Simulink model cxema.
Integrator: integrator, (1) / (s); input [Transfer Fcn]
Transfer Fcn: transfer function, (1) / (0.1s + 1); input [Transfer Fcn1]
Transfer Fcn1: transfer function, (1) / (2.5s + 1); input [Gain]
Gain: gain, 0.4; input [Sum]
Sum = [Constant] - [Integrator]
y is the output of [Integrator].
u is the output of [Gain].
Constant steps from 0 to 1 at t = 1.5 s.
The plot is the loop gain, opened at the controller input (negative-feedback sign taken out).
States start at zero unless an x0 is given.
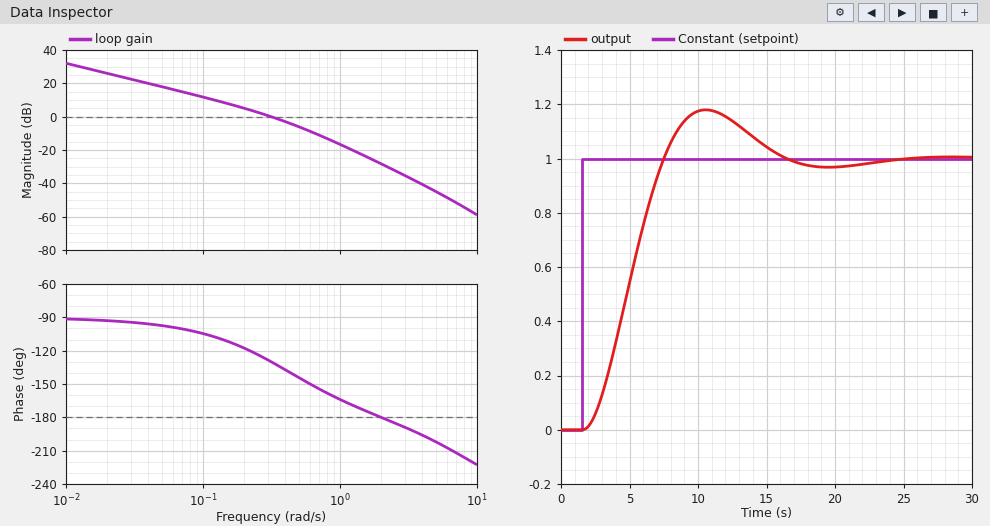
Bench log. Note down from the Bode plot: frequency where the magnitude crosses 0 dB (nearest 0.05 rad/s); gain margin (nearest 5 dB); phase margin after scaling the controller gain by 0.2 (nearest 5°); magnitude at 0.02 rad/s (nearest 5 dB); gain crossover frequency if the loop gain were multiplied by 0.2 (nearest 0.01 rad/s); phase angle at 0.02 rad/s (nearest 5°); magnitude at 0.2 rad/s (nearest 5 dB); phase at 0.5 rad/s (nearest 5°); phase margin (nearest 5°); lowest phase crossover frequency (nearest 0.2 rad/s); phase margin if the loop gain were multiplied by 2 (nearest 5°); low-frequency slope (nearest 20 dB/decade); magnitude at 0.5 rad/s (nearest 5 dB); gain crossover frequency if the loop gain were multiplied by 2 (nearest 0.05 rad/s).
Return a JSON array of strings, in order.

["0.30 rad/s", "30 dB", "80°", "25 dB", "0.08 rad/s", "-95°", "5 dB", "-145°", "50°", "2.0 rad/s", "35°", "-20 dB/decade", "-5 dB", "0.50 rad/s"]
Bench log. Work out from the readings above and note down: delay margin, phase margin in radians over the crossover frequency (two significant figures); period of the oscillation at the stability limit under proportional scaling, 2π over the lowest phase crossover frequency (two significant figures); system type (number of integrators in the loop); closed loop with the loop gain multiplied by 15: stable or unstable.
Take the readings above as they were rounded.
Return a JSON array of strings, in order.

["2.9 s", "3.1 s", "1", "stable"]
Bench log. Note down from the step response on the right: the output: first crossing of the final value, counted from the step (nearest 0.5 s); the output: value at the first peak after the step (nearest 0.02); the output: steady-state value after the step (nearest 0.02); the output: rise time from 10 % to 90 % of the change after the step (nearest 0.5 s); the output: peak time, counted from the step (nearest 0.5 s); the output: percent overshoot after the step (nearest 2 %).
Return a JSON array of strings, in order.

["6.0 s", "1.18", "1.00", "4.0 s", "9.0 s", "18 %"]
